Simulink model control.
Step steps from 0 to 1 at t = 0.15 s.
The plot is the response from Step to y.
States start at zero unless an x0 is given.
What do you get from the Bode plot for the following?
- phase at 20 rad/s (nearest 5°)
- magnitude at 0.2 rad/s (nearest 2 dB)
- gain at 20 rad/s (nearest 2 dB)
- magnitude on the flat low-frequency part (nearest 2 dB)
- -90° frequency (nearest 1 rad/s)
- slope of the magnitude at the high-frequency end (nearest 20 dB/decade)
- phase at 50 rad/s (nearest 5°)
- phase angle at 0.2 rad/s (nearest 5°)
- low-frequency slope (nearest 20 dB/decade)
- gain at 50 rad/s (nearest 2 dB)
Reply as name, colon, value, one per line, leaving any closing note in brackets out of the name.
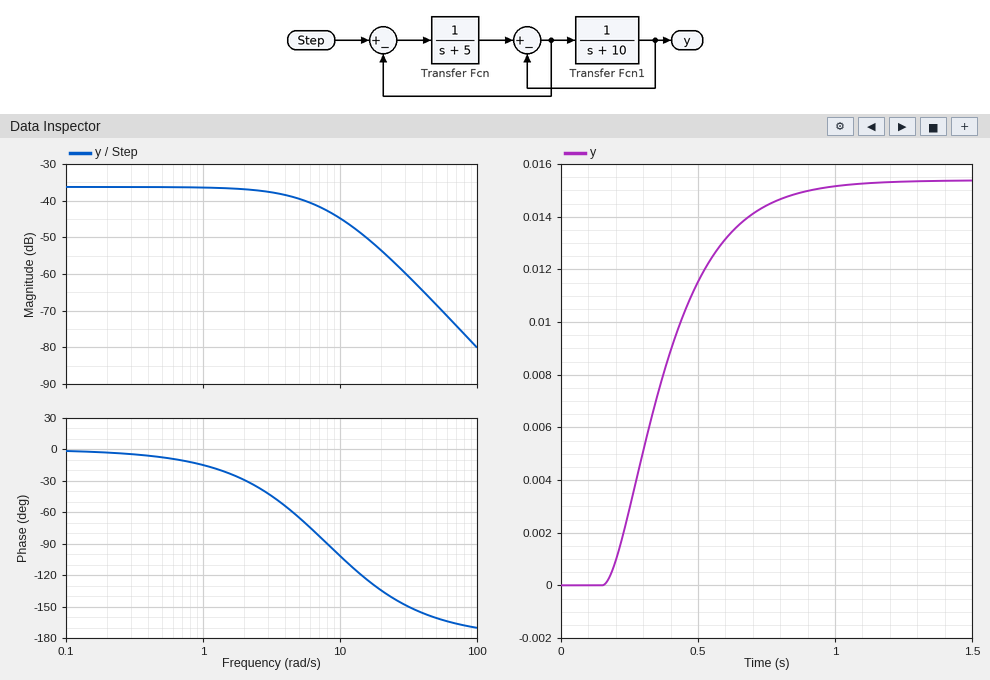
phase at 20 rad/s: -135°
magnitude at 0.2 rad/s: -36 dB
gain at 20 rad/s: -54 dB
magnitude on the flat low-frequency part: -36 dB
-90° frequency: 8 rad/s
slope of the magnitude at the high-frequency end: -40 dB/decade
phase at 50 rad/s: -160°
phase angle at 0.2 rad/s: -5°
low-frequency slope: 0 dB/decade
gain at 50 rad/s: -68 dB
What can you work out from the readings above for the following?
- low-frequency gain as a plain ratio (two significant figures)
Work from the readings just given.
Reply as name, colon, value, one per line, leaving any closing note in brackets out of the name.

low-frequency gain as a plain ratio: 0.016
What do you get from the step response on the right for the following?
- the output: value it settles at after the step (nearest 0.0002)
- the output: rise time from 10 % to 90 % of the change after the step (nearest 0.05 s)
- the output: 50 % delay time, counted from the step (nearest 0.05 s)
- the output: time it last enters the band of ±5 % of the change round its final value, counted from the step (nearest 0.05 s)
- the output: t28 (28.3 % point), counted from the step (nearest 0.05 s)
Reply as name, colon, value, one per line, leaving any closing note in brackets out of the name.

the output: value it settles at after the step: 0.0154
the output: rise time from 10 % to 90 % of the change after the step: 0.45 s
the output: 50 % delay time, counted from the step: 0.20 s
the output: time it last enters the band of ±5 % of the change round its final value, counted from the step: 0.65 s
the output: t28 (28.3 % point), counted from the step: 0.15 s
